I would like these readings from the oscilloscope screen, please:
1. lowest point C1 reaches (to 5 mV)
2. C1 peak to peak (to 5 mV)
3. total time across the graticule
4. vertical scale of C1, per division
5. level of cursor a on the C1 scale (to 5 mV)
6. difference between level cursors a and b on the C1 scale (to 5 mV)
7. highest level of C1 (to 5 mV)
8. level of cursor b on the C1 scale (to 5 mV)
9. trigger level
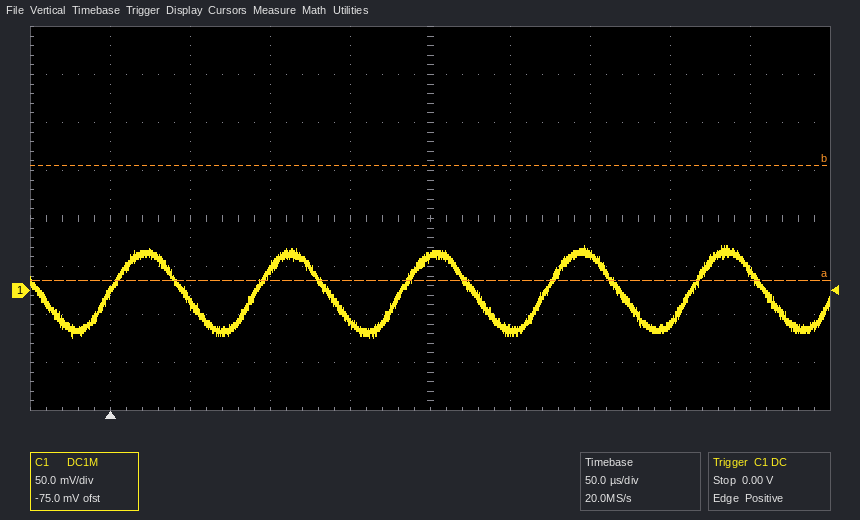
-50 mV
95 mV
500 µs
50 mV
10 mV
120 mV
45 mV
130 mV
0.00 V
